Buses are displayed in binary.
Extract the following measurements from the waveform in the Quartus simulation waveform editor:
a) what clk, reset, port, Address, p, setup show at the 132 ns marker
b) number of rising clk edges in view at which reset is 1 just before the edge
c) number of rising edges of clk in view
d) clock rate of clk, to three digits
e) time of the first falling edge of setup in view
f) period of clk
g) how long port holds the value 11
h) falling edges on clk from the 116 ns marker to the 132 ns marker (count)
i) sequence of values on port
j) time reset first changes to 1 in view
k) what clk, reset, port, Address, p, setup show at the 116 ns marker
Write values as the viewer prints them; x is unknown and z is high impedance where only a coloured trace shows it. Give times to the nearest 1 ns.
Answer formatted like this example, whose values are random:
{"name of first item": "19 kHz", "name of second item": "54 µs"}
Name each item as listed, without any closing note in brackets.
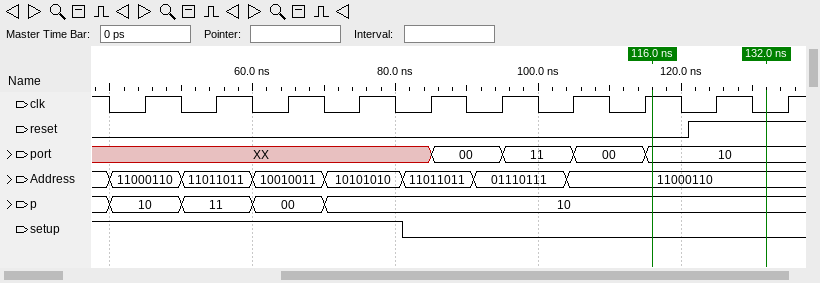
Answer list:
{"what clk, reset, port, Address, p, setup show at the 132 ns marker": "clk=0, reset=1, port=10, Address=11000110, p=10, setup=0", "number of rising clk edges in view at which reset is 1 just before the edge": "2", "number of rising edges of clk in view": "10", "clock rate of clk, to three digits": "100 MHz", "time of the first falling edge of setup in view": "81 ns", "period of clk": "10 ns", "how long port holds the value 11": "10 ns", "falling edges on clk from the 116 ns marker to the 132 ns marker": "2", "sequence of values on port": "XX, 00, 11, 00, 10", "time reset first changes to 1 in view": "121 ns", "what clk, reset, port, Address, p, setup show at the 116 ns marker": "clk=1, reset=0, port=10, Address=11000110, p=10, setup=0"}
